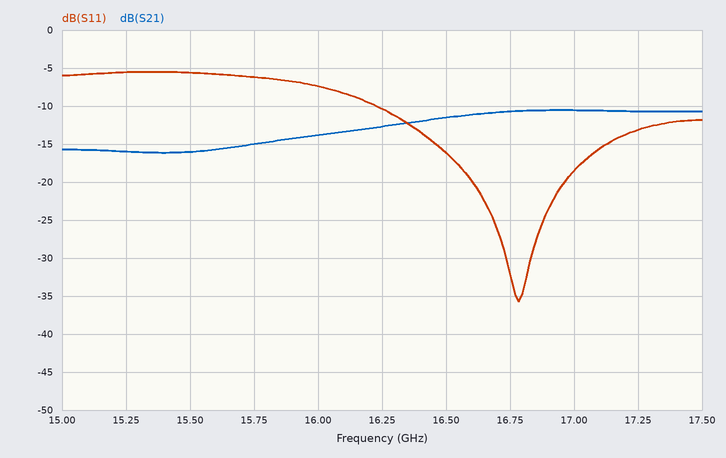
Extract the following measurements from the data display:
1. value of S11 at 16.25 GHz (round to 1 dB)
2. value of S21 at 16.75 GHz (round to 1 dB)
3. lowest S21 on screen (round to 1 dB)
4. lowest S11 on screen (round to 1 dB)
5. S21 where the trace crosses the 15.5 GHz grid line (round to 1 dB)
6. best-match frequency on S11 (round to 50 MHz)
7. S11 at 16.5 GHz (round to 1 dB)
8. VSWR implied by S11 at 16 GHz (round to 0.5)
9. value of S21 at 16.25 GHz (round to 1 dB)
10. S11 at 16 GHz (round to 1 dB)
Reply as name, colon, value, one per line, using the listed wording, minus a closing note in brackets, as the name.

value of S11 at 16.25 GHz: -10 dB
value of S21 at 16.75 GHz: -11 dB
lowest S21 on screen: -16 dB
lowest S11 on screen: -36 dB
S21 where the trace crosses the 15.5 GHz grid line: -16 dB
best-match frequency on S11: 16.80 GHz
S11 at 16.5 GHz: -16 dB
VSWR implied by S11 at 16 GHz: 2.5
value of S21 at 16.25 GHz: -13 dB
S11 at 16 GHz: -7 dB
